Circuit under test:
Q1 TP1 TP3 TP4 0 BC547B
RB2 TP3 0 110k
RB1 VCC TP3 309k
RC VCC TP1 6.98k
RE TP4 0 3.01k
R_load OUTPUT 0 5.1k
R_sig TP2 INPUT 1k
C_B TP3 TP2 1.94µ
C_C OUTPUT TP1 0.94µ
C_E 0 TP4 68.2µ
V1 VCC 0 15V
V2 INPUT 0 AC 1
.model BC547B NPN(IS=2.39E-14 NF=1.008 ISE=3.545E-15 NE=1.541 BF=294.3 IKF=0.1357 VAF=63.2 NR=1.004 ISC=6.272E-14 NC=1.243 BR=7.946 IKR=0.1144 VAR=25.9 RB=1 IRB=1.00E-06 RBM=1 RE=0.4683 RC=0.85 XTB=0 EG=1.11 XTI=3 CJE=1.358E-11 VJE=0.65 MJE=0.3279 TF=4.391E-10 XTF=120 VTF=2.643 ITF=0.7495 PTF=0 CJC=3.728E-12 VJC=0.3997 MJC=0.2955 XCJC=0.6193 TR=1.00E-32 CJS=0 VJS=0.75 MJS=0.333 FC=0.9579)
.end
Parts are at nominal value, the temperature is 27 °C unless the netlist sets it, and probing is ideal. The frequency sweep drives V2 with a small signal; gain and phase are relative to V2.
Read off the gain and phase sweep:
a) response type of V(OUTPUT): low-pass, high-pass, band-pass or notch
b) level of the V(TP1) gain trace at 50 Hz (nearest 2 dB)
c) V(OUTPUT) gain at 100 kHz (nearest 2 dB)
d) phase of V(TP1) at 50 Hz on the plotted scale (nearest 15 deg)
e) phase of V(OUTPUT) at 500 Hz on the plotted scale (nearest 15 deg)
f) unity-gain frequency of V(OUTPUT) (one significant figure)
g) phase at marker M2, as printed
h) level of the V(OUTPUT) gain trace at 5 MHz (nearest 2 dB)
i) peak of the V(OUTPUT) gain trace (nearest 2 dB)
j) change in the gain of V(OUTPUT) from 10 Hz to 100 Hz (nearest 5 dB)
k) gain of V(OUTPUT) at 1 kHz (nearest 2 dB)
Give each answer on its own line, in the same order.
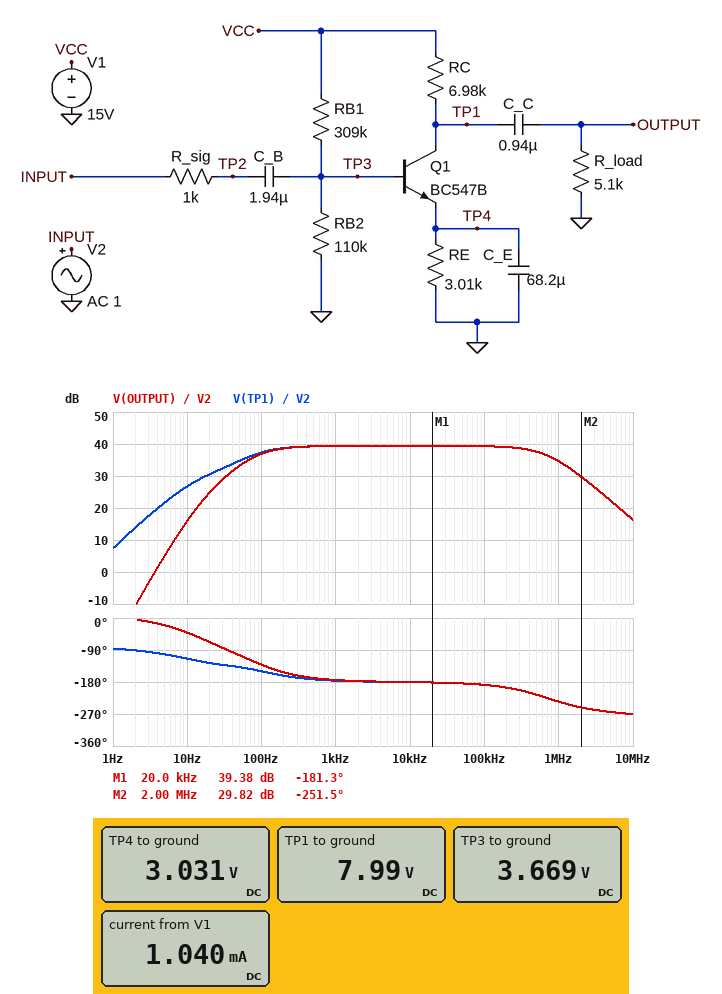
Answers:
band-pass
34 dB
40 dB
-135 deg
-165 deg
4 Hz
-251.5 deg
22 dB
40 dB
20 dB
40 dB
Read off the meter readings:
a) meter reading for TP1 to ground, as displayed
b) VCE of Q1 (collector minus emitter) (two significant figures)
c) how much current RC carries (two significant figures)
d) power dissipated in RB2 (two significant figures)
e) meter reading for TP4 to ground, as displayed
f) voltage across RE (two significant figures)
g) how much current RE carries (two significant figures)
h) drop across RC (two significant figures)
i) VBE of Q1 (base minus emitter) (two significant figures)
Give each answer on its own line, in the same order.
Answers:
7.99 V
5.0 V
1.0 mA
120 µW
3.031 V
3.0 V
1.0 mA
7.0 V
640 mV
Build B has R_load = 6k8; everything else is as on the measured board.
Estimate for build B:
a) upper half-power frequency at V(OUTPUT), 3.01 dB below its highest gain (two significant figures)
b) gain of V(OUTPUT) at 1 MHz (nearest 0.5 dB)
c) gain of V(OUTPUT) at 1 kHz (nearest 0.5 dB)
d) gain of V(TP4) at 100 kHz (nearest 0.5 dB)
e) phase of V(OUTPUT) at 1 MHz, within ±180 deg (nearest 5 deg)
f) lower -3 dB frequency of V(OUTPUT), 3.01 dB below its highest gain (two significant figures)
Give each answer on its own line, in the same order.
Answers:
630 kHz
35.0 dB
40.5 dB
-63.0 dB
120 deg
86 Hz
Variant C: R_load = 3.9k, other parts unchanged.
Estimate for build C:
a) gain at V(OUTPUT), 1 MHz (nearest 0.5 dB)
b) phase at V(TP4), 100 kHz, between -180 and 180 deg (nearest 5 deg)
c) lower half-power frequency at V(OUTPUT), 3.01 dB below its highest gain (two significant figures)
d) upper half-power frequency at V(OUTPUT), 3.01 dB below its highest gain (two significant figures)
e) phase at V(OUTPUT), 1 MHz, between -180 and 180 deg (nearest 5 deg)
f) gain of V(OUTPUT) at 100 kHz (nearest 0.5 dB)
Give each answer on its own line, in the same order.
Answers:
34.0 dB
-95 deg
89 Hz
790 kHz
130 deg
38.0 dB
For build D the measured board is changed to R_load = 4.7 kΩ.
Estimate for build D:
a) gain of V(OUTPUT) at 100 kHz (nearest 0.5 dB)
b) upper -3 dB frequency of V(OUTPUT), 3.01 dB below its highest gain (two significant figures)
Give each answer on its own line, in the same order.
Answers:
39.0 dB
730 kHz
